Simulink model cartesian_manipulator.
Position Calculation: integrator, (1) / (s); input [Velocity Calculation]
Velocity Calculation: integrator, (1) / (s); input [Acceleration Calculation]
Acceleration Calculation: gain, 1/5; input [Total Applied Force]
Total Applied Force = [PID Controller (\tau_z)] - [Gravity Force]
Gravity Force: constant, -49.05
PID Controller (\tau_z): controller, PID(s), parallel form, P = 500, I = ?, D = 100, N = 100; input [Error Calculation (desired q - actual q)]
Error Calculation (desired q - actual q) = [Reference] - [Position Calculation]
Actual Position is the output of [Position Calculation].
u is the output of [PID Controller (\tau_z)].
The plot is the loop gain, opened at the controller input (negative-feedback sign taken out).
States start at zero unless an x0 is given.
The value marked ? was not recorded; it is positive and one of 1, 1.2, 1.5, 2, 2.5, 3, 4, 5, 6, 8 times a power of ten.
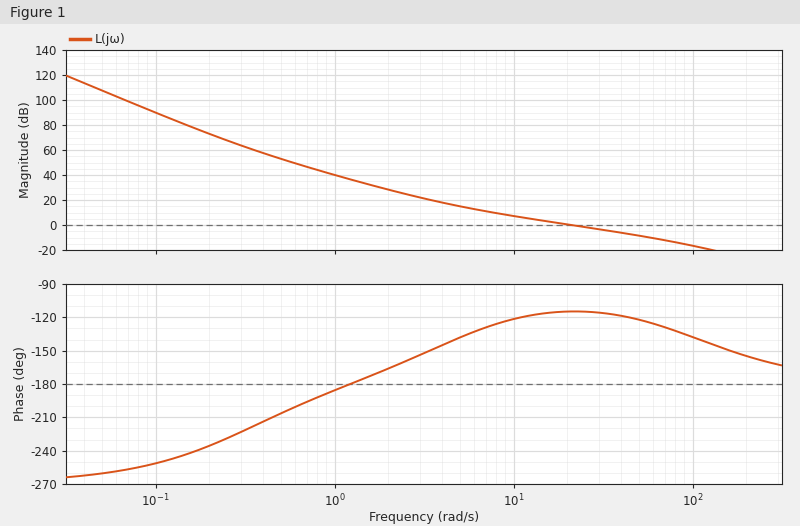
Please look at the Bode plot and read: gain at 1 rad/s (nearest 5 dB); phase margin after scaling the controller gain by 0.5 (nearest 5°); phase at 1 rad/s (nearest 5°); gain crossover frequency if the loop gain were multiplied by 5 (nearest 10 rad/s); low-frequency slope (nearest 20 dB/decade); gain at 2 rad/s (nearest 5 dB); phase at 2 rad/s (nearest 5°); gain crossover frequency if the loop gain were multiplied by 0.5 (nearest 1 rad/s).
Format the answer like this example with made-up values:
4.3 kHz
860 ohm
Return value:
40 dB
60°
-185°
80 rad/s
-60 dB/decade
30 dB
-165°
11 rad/s
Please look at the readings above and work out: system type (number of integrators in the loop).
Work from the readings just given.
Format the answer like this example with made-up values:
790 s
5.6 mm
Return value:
3
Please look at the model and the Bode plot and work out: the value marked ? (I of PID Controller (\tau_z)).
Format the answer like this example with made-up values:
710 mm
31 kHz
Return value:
150
